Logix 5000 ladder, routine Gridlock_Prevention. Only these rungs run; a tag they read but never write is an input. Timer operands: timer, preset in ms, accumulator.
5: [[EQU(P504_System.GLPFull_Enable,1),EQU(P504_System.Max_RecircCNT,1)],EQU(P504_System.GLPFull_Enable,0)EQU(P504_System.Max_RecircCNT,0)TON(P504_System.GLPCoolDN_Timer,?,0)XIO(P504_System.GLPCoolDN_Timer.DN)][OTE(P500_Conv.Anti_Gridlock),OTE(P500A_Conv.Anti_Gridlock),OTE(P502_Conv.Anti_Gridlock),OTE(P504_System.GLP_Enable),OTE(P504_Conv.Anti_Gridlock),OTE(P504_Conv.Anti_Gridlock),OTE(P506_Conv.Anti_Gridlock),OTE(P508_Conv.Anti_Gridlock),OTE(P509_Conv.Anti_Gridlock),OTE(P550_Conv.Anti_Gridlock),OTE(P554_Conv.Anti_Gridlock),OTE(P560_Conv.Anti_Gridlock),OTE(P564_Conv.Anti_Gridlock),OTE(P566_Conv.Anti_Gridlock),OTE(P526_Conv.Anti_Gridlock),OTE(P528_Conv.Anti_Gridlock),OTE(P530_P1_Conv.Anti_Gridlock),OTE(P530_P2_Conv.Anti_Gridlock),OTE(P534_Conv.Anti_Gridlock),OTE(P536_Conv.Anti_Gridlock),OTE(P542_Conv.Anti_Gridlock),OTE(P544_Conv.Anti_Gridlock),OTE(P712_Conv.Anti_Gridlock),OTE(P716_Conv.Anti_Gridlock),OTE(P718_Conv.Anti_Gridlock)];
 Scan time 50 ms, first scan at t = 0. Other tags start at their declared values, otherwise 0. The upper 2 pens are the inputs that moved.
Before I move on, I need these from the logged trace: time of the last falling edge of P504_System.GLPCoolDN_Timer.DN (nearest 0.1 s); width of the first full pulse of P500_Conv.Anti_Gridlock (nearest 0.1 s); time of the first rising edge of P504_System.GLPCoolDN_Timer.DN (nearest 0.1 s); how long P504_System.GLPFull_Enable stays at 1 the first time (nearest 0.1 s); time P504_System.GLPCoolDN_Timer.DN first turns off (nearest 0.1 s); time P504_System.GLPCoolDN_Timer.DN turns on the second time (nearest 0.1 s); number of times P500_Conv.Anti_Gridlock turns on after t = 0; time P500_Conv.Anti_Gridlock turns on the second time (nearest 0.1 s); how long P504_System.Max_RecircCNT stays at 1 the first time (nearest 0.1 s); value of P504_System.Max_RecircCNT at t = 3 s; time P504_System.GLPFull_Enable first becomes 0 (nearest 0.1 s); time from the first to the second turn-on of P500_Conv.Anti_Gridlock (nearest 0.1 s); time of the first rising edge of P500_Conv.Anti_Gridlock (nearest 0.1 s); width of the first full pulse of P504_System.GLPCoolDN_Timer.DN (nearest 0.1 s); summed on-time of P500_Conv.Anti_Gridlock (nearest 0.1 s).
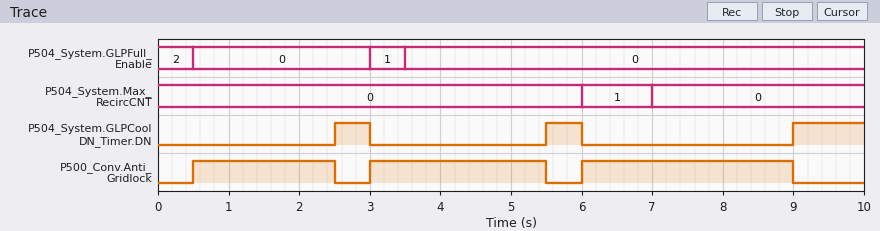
6.0 s
2.0 s
2.5 s
0.5 s
3.0 s
5.5 s
3
3.0 s
1.0 s
0
0.5 s
2.5 s
0.5 s
0.5 s
7.5 s
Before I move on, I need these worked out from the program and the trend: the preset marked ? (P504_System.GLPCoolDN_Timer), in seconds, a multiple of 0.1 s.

2.0 s
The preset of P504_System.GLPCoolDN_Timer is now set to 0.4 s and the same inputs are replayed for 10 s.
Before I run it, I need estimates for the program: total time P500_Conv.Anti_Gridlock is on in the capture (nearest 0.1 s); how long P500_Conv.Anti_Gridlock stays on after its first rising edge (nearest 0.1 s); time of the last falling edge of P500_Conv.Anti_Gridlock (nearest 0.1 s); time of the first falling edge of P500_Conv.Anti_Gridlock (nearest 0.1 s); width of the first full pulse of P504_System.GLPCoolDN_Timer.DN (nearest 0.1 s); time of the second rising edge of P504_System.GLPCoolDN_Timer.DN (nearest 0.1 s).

2.7 s
0.4 s
7.4 s
0.9 s
2.1 s
3.9 s
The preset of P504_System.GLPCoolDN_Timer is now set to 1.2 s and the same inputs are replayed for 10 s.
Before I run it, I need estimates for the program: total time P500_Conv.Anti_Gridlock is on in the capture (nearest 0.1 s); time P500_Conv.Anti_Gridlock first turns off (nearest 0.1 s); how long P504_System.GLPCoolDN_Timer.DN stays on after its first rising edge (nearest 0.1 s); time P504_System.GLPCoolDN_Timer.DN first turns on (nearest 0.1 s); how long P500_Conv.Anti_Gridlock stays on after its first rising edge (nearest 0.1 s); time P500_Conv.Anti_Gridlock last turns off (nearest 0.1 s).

5.1 s
1.7 s
1.3 s
1.7 s
1.2 s
8.2 s
